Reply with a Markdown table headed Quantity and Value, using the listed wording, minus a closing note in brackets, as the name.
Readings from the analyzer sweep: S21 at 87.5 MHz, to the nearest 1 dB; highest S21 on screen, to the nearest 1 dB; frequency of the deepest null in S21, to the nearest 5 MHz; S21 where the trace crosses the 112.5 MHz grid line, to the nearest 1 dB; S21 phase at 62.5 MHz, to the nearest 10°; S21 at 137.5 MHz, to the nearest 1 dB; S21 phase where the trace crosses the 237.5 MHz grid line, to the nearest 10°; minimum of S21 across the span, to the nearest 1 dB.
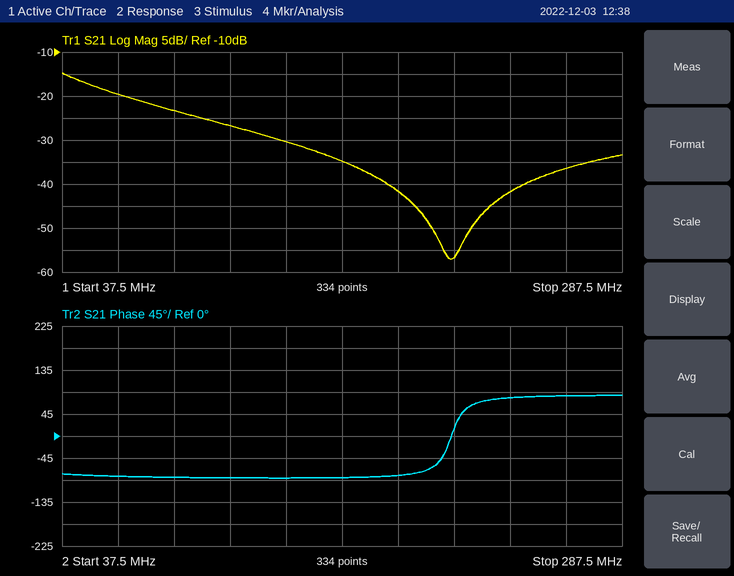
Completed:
| Quantity | Value |
|---|---|
| S21 at 87.5 MHz, to the nearest 1 dB | -23 dB |
| highest S21 on screen, to the nearest 1 dB | -15 dB |
| frequency of the deepest null in S21, to the nearest 5 MHz | 210 MHz |
| S21 where the trace crosses the 112.5 MHz grid line, to the nearest 1 dB | -27 dB |
| S21 phase at 62.5 MHz, to the nearest 10° | -80° |
| S21 at 137.5 MHz, to the nearest 1 dB | -30 dB |
| S21 phase where the trace crosses the 237.5 MHz grid line, to the nearest 10° | 80° |
| minimum of S21 across the span, to the nearest 1 dB | -57 dB |
